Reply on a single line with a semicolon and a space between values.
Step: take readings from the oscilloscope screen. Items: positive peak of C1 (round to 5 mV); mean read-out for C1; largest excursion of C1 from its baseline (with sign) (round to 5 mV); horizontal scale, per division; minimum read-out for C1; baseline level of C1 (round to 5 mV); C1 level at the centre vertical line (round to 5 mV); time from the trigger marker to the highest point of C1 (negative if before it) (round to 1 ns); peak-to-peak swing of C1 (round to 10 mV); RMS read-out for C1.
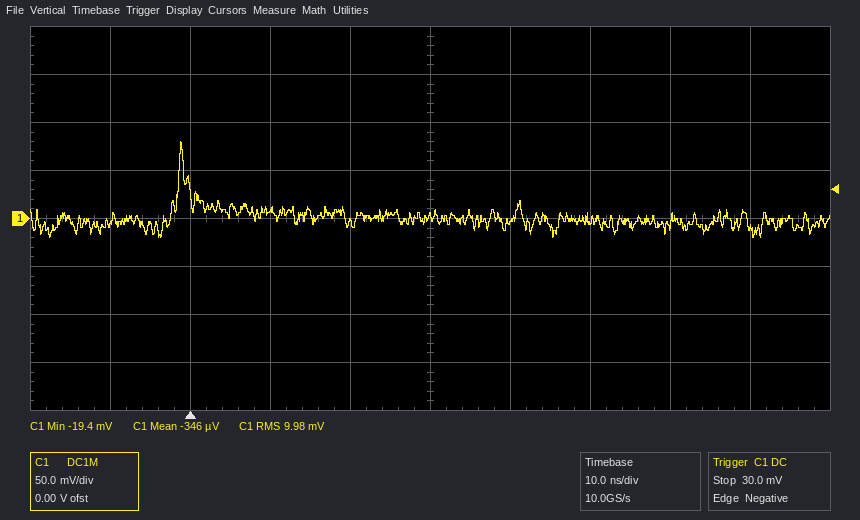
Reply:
80 mV; -346 µV; +80 mV; 10 ns; -19.4 mV; 0 mV; 0 mV; -1 ns; 100 mV; 9.98 mV
